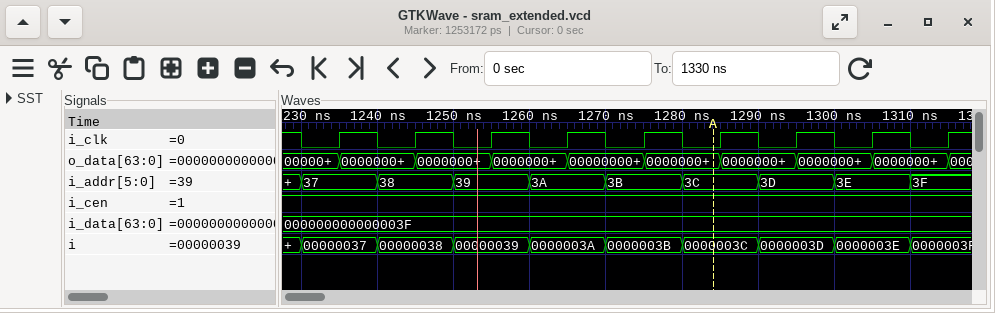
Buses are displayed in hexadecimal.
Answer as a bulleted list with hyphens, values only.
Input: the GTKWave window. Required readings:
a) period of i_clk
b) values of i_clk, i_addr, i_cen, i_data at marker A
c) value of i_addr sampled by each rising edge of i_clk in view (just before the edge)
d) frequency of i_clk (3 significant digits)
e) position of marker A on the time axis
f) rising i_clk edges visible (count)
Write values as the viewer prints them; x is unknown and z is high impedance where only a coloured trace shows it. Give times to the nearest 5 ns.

- 10 ns
- i_clk=0, i_addr=3C, i_cen=1, i_data=000000000000003F
- 37, 38, 39, 3A, 3B, 3C, 3D, 3E, 3F
- 100 MHz
- 1285 ns
- 9
